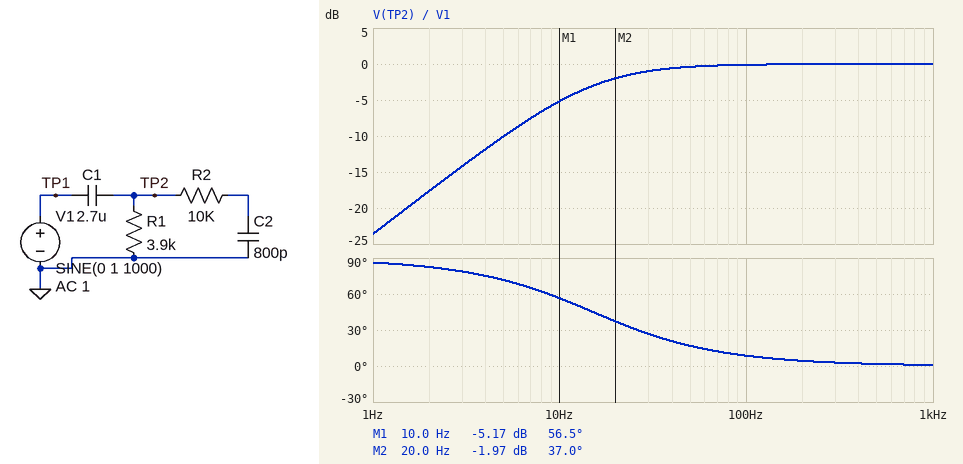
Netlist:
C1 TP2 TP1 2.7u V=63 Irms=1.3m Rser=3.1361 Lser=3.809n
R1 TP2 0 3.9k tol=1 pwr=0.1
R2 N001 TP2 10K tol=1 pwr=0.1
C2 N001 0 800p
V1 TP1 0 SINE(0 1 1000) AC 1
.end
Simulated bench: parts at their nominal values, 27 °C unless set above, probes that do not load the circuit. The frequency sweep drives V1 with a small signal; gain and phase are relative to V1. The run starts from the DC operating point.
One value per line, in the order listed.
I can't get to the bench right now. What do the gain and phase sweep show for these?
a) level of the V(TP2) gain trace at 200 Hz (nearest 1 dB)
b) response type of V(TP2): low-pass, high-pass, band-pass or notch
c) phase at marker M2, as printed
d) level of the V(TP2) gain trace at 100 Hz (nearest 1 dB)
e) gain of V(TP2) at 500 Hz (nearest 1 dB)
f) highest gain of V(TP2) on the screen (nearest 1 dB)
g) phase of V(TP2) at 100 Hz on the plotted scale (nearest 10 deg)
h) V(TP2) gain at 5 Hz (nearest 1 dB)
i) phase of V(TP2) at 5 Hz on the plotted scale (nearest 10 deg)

0 dB
high-pass
37.0 deg
0 dB
0 dB
0 dB
10 deg
-10 dB
70 deg
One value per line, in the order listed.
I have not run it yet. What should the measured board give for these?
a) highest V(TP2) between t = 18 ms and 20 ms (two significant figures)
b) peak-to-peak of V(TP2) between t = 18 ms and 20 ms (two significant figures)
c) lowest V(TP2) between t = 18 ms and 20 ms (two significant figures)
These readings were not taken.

1.0 V
2.0 V
-1.0 V
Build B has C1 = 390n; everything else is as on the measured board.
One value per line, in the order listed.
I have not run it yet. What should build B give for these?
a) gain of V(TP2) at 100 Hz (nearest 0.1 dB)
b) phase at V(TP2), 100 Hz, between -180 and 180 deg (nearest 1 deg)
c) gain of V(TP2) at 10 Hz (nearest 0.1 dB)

-3.2 dB
46 deg
-20.4 dB
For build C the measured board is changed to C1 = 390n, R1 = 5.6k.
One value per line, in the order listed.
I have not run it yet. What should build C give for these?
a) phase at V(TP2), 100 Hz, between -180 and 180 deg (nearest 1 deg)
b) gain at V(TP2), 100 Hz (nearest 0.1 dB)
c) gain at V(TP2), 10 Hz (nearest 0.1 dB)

36 deg
-1.9 dB
-17.3 dB
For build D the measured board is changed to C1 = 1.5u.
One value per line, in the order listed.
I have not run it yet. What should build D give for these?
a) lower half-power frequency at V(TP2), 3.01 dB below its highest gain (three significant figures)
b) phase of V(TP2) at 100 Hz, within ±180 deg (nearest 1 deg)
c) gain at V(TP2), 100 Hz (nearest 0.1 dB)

27.2 Hz
15 deg
-0.3 dB
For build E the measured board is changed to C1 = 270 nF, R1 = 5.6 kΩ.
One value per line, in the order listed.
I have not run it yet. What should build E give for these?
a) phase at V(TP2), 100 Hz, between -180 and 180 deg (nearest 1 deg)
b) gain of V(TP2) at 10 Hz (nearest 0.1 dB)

46 deg
-20.5 dB
